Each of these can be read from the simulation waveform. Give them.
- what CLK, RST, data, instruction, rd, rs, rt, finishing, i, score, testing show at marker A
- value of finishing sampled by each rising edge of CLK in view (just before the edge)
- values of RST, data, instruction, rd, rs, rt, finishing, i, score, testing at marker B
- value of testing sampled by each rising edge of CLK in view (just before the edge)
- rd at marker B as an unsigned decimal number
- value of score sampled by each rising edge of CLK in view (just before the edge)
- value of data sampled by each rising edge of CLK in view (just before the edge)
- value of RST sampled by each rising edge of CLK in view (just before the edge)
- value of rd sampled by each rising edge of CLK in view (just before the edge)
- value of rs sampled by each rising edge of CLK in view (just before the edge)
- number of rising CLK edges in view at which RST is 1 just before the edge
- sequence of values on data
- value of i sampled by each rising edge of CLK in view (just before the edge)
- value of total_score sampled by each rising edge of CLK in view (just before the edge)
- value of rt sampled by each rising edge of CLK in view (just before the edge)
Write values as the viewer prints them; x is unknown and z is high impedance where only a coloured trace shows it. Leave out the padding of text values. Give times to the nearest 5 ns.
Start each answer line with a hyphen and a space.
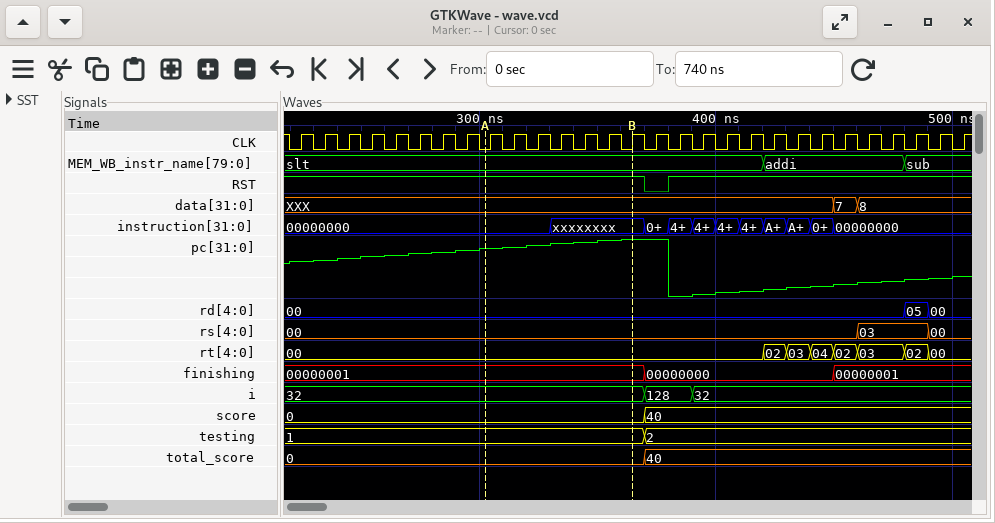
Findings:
- CLK=0, RST=1, data=XXX, instruction=00000000, rd=00, rs=00, rt=00, finishing=00000001, i=32, score=0, testing=1
- 00000001, 00000001, 00000001, 00000001, 00000001, 00000001, 00000001, 00000001, 00000001, 00000001, 00000001, 00000001, 00000001, 00000001, 00000001, 00000000, 00000000, 00000000, 00000000, 00000000, 00000000, 00000000, 00000000, 00000001, 00000001, 00000001, 00000001, 00000001, 00000001
- RST=1, data=XXX, instruction=xxxxxxxx, rd=00, rs=00, rt=00, finishing=00000001, i=32, score=0, testing=1
- 1, 1, 1, 1, 1, 1, 1, 1, 1, 1, 1, 1, 1, 1, 1, 2, 2, 2, 2, 2, 2, 2, 2, 2, 2, 2, 2, 2, 2
- 0
- 0, 0, 0, 0, 0, 0, 0, 0, 0, 0, 0, 0, 0, 0, 0, 40, 40, 40, 40, 40, 40, 40, 40, 40, 40, 40, 40, 40, 40
- XXX, XXX, XXX, XXX, XXX, XXX, XXX, XXX, XXX, XXX, XXX, XXX, XXX, XXX, XXX, XXX, XXX, XXX, XXX, XXX, XXX, XXX, XXX, 7, 8, 8, 8, 8, 8
- 1 1 1 1 1 1 1 1 1 1 1 1 1 1 1 0 1 1 1 1 1 1 1 1 1 1 1 1 1
- 00, 00, 00, 00, 00, 00, 00, 00, 00, 00, 00, 00, 00, 00, 00, 00, 00, 00, 00, 00, 00, 00, 00, 00, 00, 00, 05, 00, 00
- 00, 00, 00, 00, 00, 00, 00, 00, 00, 00, 00, 00, 00, 00, 00, 00, 00, 00, 00, 00, 00, 00, 00, 00, 03, 03, 03, 00, 00
- 28
- XXX, 7, 8
- 32, 32, 32, 32, 32, 32, 32, 32, 32, 32, 32, 32, 32, 32, 32, 128, 128, 32, 32, 32, 32, 32, 32, 32, 32, 32, 32, 32, 32
- 0, 0, 0, 0, 0, 0, 0, 0, 0, 0, 0, 0, 0, 0, 0, 40, 40, 40, 40, 40, 40, 40, 40, 40, 40, 40, 40, 40, 40
- 00, 00, 00, 00, 00, 00, 00, 00, 00, 00, 00, 00, 00, 00, 00, 00, 00, 00, 00, 00, 02, 03, 04, 02, 03, 03, 02, 00, 00
